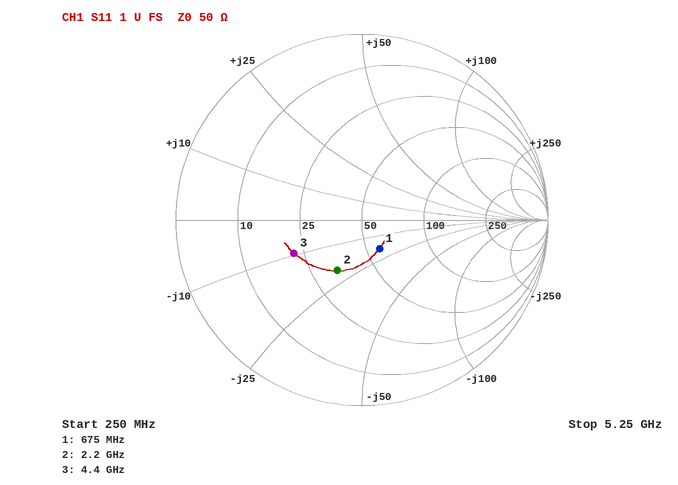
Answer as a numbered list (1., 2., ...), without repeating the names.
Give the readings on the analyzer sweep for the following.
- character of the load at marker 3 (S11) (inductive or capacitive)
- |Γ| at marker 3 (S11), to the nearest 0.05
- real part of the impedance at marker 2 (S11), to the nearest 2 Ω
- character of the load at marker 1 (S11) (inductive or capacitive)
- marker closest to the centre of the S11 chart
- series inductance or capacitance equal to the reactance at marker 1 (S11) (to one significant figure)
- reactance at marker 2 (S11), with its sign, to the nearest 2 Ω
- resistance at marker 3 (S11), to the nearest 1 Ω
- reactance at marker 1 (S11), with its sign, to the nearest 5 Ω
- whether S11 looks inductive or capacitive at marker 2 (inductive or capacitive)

1. capacitive
2. 0.40
3. 34 Ω
4. capacitive
5. marker 1
6. 10 pF
7. -20 Ω
8. 22 Ω
9. -20 Ω
10. capacitive
